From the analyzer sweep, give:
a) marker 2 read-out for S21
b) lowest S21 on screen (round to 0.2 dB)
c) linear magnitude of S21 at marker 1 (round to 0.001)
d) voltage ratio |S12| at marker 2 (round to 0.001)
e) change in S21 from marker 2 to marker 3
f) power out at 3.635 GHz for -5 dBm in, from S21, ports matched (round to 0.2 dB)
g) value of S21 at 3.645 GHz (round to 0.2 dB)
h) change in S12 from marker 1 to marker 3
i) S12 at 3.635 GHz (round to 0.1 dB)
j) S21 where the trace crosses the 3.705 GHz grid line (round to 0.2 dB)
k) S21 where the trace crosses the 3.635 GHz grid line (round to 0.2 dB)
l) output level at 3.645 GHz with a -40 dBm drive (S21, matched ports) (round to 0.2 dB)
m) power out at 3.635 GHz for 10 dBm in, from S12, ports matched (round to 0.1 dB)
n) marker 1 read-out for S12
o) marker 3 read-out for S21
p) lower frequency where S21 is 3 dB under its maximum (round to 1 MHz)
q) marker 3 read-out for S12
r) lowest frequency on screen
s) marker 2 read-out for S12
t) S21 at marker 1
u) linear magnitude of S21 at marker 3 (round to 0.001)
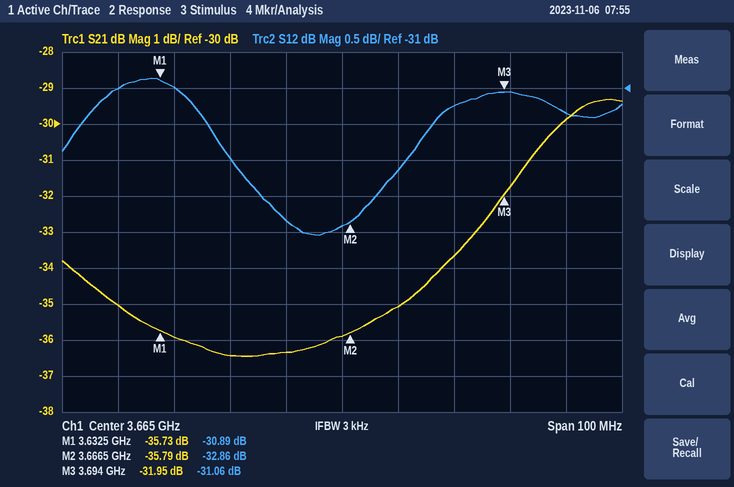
-35.79 dB
-36.4 dB
0.016
0.023
3.84 dB
-41.0 dBm
-36.4 dB
-0.17 dB
-31.0 dB
-29.8 dB
-36.0 dB
-76.4 dBm
-21.0 dBm
-30.89 dB
-31.95 dB
3.692 GHz
-31.06 dB
3.615 GHz
-32.86 dB
-35.73 dB
0.025
